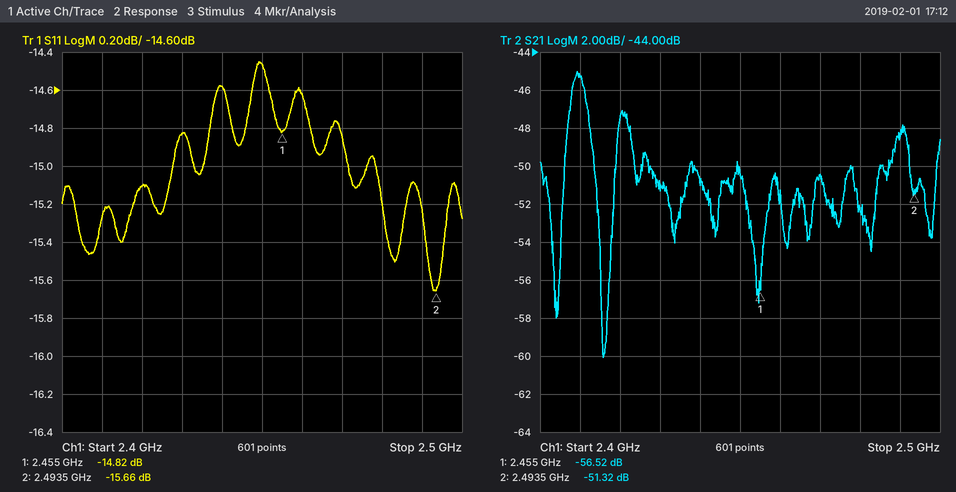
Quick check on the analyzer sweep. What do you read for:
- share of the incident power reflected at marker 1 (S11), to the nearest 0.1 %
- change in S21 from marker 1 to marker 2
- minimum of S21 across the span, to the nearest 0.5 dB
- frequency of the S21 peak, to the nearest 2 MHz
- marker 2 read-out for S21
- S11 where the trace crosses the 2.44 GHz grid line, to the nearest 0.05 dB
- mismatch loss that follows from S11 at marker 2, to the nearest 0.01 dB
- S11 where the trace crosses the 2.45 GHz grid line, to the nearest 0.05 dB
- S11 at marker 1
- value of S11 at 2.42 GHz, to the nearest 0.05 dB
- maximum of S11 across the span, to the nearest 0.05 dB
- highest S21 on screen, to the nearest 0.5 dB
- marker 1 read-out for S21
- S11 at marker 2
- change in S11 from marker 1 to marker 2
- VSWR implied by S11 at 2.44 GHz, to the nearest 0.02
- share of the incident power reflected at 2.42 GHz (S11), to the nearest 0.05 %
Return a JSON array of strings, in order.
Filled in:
["3.3 %", "5.20 dB", "-60.0 dB", "2.410 GHz", "-51.32 dB", "-14.60 dB", "0.12 dB", "-14.45 dB", "-14.82 dB", "-15.10 dB", "-14.45 dB", "-45.0 dB", "-56.52 dB", "-15.66 dB", "-0.84 dB", "1.46", "3.10 %"]
